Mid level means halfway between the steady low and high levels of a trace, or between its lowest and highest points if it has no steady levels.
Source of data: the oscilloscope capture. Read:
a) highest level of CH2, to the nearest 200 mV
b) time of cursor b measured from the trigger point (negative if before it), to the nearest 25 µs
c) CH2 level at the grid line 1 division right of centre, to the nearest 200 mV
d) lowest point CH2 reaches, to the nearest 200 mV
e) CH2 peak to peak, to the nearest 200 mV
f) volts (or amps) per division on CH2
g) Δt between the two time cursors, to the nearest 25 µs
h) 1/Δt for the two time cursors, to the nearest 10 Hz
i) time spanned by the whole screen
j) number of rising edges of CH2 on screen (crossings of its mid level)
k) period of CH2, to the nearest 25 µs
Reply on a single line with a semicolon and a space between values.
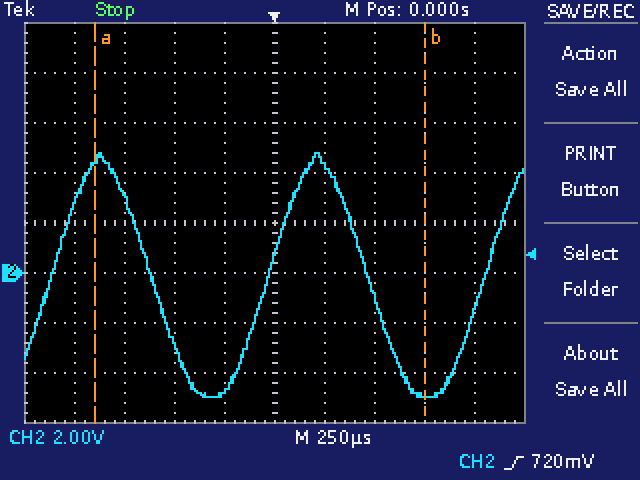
4.8 V; +750 µs; 4.4 V; -5.0 V; 9.8 V; 2 V; 1.650 ms; 610 Hz; 2.5 ms; 3; 1.075 ms
